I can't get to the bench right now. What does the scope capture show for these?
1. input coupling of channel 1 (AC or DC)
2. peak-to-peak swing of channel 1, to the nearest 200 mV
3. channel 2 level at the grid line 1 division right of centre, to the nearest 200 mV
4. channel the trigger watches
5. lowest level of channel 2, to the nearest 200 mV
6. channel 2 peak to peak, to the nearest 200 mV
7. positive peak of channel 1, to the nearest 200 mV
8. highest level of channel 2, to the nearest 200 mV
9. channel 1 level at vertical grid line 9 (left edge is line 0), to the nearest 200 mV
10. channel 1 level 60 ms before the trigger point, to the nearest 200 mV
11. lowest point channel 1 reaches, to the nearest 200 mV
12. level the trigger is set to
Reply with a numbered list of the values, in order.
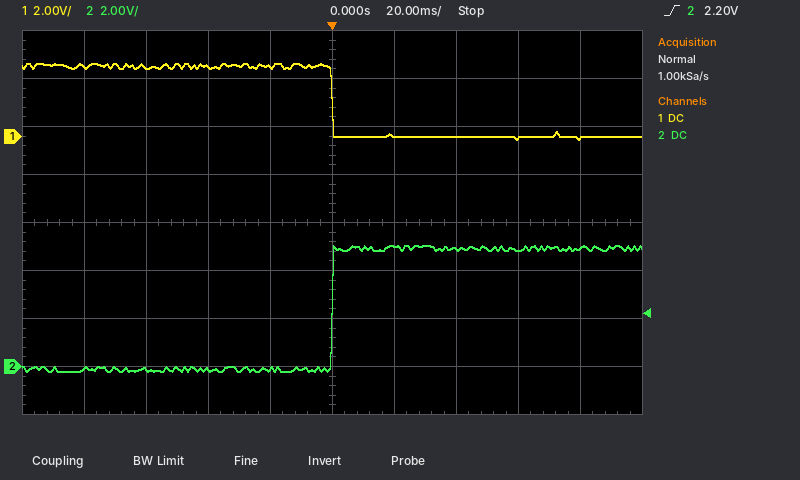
1. DC
2. 3.2 V
3. 5.0 V
4. channel 2
5. -200 mV
6. 5.2 V
7. 3.0 V
8. 5.0 V
9. 0.0 V
10. 2.8 V
11. -200 mV
12. 2.20 V
